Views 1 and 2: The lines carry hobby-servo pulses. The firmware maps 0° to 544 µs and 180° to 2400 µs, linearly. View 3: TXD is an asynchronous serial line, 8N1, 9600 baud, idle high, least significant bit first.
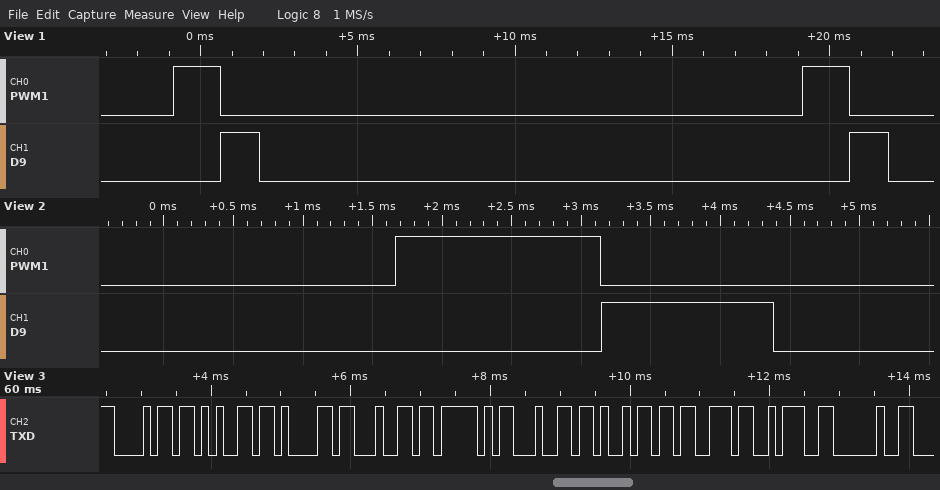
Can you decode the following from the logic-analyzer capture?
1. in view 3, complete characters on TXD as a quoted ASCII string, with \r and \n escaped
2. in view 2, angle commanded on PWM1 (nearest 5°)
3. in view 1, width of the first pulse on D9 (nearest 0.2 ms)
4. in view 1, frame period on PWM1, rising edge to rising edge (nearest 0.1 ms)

"head_dis: "
90°
1.2 ms
20.0 ms
